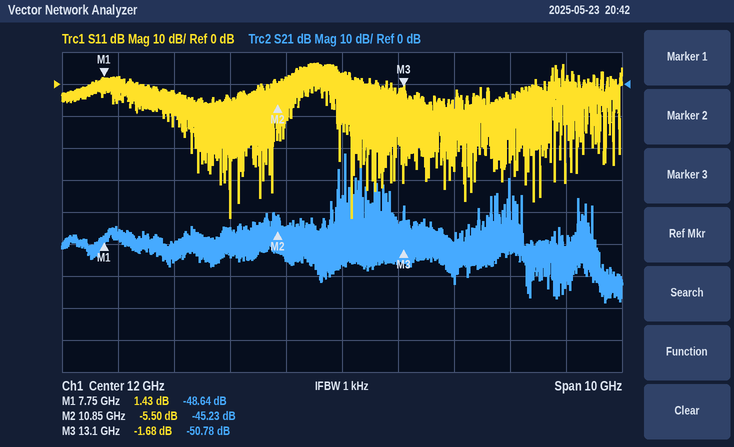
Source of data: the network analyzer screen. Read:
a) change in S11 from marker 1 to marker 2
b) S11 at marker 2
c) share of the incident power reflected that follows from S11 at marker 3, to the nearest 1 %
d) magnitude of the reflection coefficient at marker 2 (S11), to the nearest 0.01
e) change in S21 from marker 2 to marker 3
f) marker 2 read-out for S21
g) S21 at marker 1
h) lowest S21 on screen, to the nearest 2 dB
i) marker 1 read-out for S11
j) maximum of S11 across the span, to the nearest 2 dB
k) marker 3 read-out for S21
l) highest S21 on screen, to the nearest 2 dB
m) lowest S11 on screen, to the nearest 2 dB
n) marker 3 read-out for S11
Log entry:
-6.93 dB
-5.50 dB
68 %
0.53
-5.55 dB
-45.23 dB
-48.64 dB
-68 dB
1.43 dB
6 dB
-50.78 dB
-22 dB
-42 dB
-1.68 dB
